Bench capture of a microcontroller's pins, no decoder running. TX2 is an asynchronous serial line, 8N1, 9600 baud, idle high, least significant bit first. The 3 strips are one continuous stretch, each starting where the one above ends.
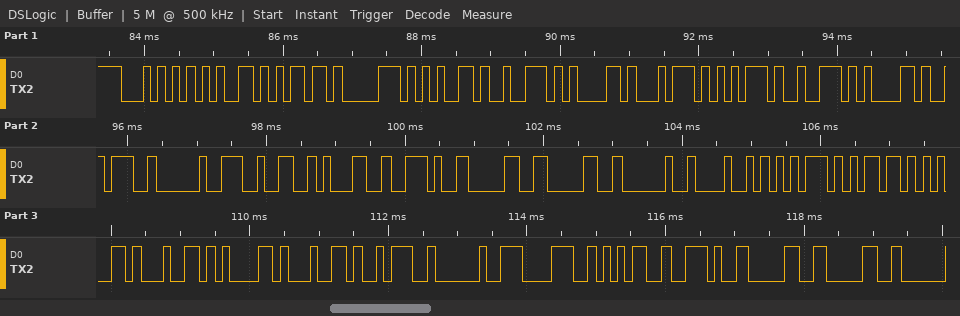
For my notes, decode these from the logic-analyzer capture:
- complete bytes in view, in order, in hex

54 65 6D 70 65 72 61 74 75 72 61 3A 20 32 31 2E 30 30 20 48 75 6D 65 64 61 64 3A 20 38 35 2E 30 30
